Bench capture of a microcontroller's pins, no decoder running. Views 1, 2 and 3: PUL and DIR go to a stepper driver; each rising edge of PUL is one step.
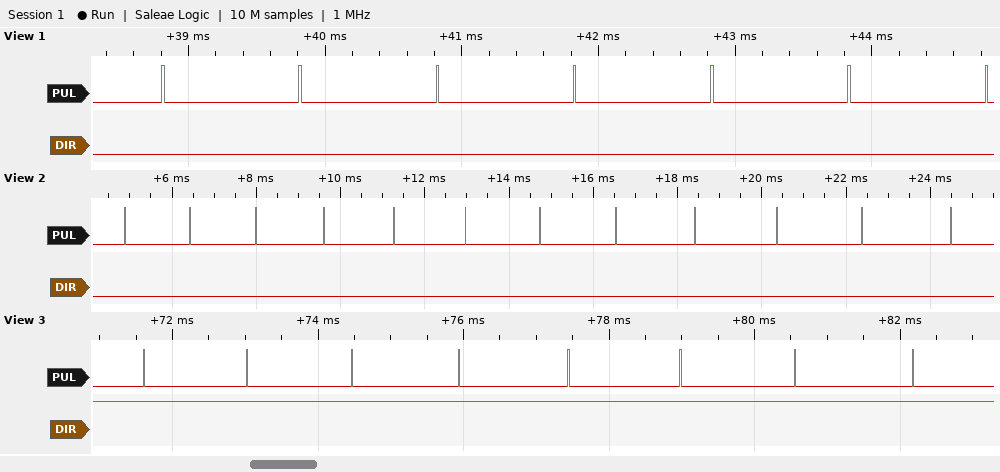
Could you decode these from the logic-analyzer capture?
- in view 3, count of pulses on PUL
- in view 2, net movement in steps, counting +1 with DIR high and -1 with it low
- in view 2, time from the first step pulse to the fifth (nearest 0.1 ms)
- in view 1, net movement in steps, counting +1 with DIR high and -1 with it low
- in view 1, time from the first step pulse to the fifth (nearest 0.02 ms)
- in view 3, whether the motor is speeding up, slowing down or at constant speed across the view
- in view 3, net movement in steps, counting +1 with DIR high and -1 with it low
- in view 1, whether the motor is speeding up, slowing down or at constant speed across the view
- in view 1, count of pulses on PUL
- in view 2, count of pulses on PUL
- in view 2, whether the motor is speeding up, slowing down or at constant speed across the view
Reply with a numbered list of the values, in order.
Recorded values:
1. 8
2. -12
3. 6.4 ms
4. -7
5. 4.02 ms
6. slowing down
7. +8
8. constant speed
9. 7
10. 12
11. slowing down
